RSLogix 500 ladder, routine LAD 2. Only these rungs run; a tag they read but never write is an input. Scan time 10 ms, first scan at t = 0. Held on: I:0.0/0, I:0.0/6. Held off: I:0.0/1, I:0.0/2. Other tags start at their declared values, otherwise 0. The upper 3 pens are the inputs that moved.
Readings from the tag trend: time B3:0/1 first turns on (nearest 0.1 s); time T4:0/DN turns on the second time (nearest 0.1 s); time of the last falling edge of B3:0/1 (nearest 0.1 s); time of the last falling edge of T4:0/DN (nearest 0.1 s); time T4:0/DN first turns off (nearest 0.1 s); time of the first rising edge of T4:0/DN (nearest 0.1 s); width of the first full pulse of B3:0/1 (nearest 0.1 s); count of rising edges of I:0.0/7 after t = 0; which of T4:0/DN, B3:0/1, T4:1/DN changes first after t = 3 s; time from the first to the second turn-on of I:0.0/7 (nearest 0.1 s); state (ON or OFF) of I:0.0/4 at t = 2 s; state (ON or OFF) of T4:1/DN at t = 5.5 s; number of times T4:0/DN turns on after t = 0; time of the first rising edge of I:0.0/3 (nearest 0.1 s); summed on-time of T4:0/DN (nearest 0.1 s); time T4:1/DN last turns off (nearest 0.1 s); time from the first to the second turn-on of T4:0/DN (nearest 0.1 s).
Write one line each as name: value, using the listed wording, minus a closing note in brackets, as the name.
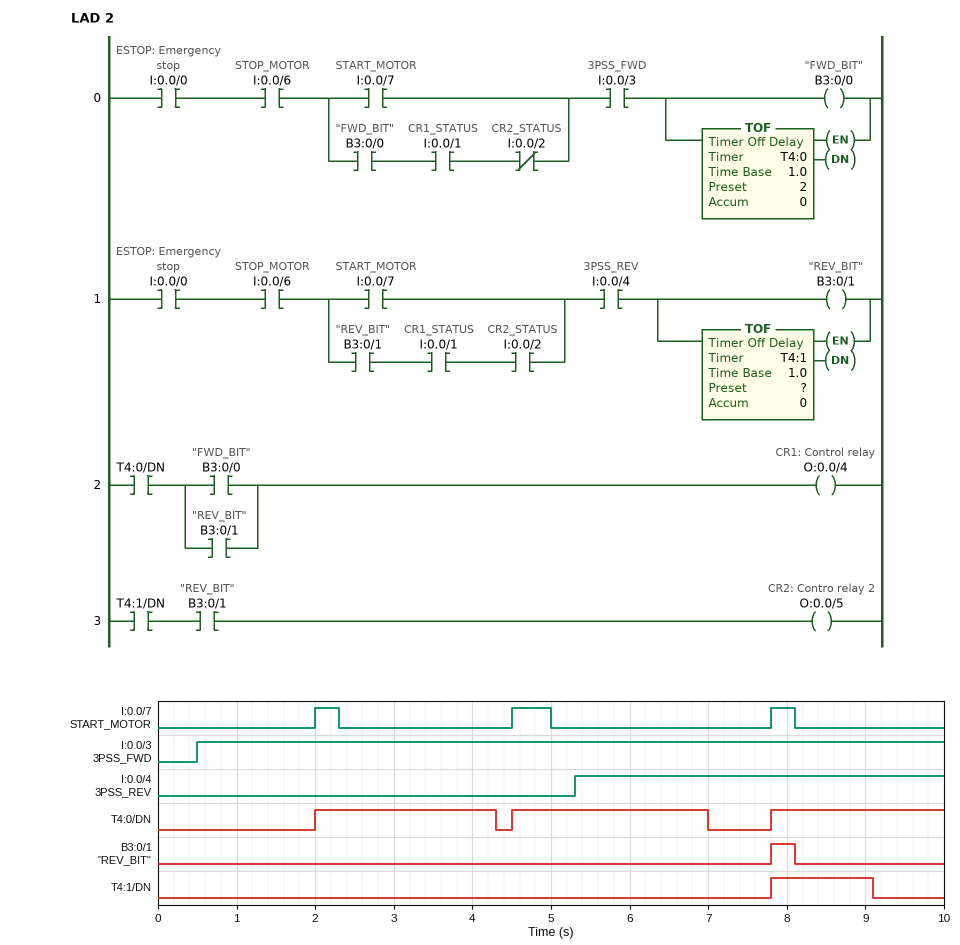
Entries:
time B3:0/1 first turns on: 7.8 s
time T4:0/DN turns on the second time: 4.5 s
time of the last falling edge of B3:0/1: 8.1 s
time of the last falling edge of T4:0/DN: 7.0 s
time T4:0/DN first turns off: 4.3 s
time of the first rising edge of T4:0/DN: 2.0 s
width of the first full pulse of B3:0/1: 0.3 s
count of rising edges of I:0.0/7 after t = 0: 3
which of T4:0/DN, B3:0/1, T4:1/DN changes first after t = 3 s: T4:0/DN
time from the first to the second turn-on of I:0.0/7: 2.5 s
state (ON or OFF) of I:0.0/4 at t = 2 s: OFF
state (ON or OFF) of T4:1/DN at t = 5.5 s: OFF
number of times T4:0/DN turns on after t = 0: 3
time of the first rising edge of I:0.0/3: 0.5 s
summed on-time of T4:0/DN: 7.0 s
time T4:1/DN last turns off: 9.1 s
time from the first to the second turn-on of T4:0/DN: 2.5 s
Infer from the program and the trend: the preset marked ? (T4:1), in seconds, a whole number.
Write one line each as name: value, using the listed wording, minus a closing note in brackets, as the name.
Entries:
the preset marked ? (T4:1), in seconds, a whole number: 1 s
